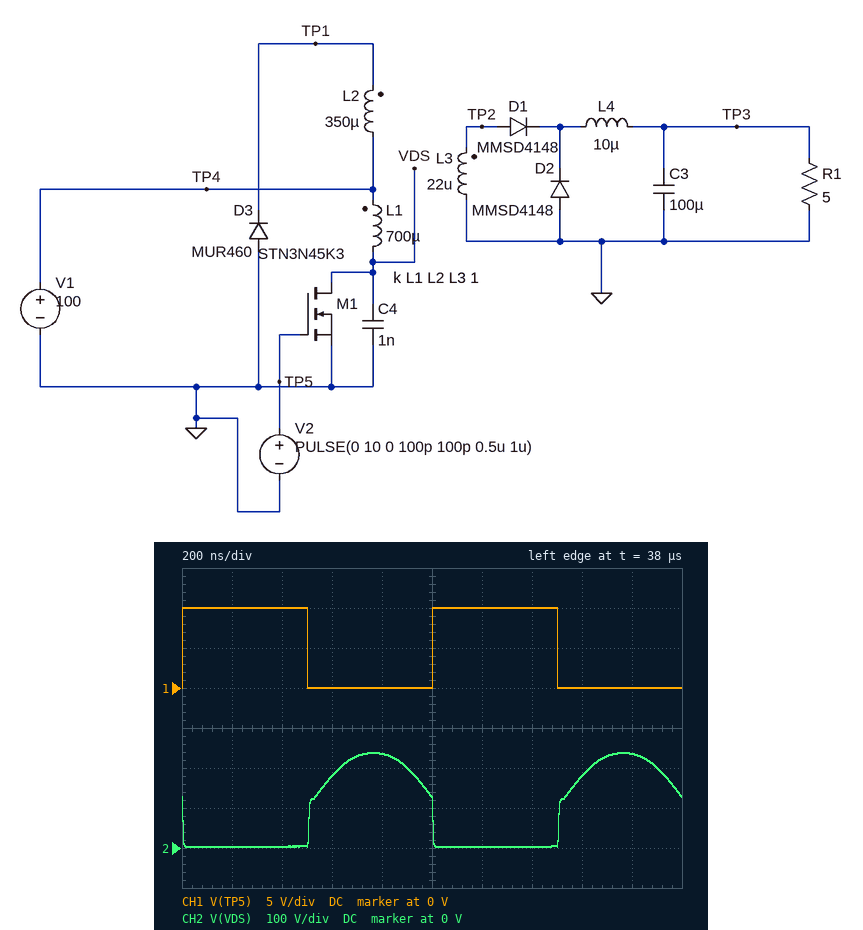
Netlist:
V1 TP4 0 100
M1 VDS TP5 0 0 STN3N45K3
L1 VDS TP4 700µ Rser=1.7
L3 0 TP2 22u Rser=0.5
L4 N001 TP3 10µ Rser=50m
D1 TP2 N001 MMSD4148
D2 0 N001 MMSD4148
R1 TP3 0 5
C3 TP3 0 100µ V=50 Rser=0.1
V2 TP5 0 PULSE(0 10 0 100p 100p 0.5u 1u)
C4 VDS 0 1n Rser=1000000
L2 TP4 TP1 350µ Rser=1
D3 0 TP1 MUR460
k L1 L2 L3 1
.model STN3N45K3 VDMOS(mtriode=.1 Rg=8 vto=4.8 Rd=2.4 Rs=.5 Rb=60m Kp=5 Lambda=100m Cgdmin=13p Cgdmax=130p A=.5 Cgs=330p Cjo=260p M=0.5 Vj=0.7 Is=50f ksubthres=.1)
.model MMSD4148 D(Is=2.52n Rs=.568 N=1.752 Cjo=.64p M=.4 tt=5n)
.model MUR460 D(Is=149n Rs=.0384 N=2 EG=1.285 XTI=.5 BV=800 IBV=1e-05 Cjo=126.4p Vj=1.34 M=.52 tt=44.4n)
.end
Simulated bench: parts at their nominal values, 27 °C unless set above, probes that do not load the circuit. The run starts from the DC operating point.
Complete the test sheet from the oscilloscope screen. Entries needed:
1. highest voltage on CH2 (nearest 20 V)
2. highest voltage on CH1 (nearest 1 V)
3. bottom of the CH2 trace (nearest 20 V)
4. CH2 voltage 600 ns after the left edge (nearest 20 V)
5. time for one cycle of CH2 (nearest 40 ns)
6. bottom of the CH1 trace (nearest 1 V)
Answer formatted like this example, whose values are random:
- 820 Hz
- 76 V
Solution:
- 240 V
- 10 V
- 0 V
- 180 V
- 1.00 µs
- 0 V
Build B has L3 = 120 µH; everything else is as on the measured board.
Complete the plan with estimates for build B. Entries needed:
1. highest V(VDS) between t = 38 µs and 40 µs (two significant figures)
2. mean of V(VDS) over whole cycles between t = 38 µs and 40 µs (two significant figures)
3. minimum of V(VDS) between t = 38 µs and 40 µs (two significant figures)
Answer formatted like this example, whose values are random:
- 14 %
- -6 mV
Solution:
- 210 V
- 96 V
- 16 V
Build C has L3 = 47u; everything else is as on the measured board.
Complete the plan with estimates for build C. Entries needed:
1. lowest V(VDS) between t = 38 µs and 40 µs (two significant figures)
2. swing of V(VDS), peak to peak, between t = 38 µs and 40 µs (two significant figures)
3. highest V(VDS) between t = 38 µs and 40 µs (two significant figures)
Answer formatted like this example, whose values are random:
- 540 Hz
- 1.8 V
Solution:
- 7.1 V
- 220 V
- 230 V
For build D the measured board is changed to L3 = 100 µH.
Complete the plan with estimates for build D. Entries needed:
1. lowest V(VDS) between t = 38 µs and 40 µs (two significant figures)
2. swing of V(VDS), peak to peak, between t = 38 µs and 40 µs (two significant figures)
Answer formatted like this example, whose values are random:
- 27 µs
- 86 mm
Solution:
- 14 V
- 200 V
